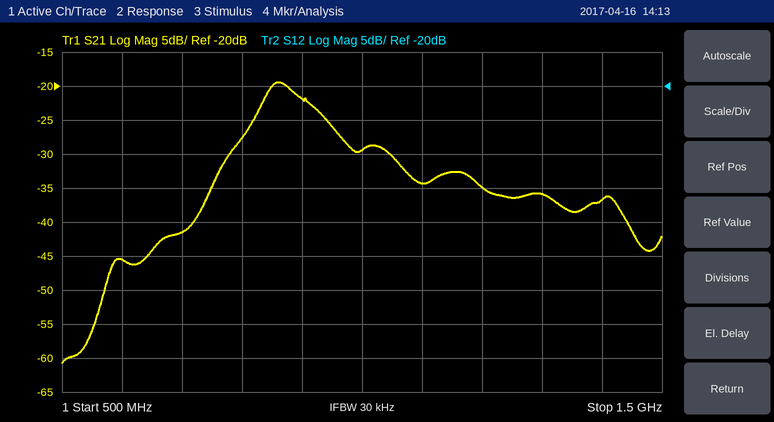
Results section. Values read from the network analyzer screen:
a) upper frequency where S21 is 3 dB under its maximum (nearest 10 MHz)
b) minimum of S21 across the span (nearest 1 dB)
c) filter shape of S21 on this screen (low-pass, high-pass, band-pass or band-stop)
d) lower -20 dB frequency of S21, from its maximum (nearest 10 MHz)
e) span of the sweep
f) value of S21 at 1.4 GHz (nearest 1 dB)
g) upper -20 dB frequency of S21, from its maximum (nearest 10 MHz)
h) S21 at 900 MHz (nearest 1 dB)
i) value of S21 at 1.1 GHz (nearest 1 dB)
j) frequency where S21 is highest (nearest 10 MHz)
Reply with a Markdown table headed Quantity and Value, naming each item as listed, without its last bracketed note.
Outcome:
| Quantity | Value |
|---|---|
| upper frequency where S21 is 3 dB under its maximum | 910 MHz |
| minimum of S21 across the span | -61 dB |
| filter shape of S21 on this screen | band-pass |
| lower -20 dB frequency of S21, from its maximum | 720 MHz |
| span of the sweep | 1 GHz |
| value of S21 at 1.4 GHz | -37 dB |
| upper -20 dB frequency of S21, from its maximum | 1.44 GHz |
| S21 at 900 MHz | -22 dB |
| value of S21 at 1.1 GHz | -34 dB |
| frequency where S21 is highest | 860 MHz |
